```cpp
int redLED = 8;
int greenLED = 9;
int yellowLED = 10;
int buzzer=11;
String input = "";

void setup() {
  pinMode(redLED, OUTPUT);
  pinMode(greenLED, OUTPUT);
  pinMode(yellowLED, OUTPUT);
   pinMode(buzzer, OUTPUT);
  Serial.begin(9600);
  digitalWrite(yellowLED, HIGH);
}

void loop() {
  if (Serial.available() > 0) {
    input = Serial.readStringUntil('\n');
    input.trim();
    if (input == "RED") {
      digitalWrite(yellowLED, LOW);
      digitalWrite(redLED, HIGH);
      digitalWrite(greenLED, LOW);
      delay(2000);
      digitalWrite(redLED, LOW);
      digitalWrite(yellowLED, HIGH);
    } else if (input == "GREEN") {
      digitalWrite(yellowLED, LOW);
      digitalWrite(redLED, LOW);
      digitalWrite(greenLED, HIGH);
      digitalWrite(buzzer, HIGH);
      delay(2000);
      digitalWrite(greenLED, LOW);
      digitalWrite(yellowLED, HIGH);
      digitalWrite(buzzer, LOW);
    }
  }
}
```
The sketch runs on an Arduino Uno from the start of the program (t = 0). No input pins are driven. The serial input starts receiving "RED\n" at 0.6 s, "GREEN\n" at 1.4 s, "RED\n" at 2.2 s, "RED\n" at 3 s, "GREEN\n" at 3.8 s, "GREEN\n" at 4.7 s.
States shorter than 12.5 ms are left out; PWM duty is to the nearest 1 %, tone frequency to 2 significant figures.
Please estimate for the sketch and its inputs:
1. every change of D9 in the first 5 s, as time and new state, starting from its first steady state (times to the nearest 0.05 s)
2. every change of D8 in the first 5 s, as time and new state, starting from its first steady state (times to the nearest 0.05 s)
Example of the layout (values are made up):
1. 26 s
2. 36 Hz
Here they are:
1. 0 s low; 2.6 s high; 4.6 s low
2. 0 s low; 0.6 s high; 2.6 s low; 4.6 s high
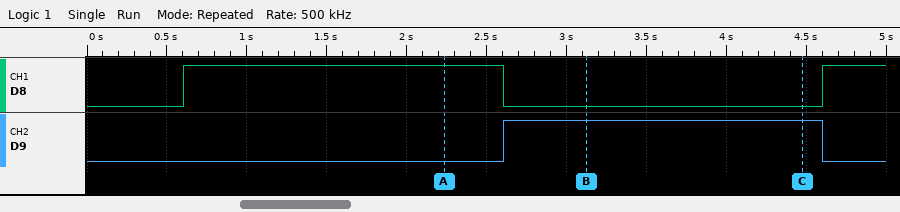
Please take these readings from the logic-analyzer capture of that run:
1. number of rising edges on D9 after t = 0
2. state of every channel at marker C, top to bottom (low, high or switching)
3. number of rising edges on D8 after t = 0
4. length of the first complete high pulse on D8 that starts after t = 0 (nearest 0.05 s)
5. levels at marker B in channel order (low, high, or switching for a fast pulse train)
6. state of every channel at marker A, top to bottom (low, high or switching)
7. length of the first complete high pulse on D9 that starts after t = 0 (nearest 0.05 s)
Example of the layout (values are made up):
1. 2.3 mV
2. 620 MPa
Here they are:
1. 1
2. D8 low, D9 high
3. 2
4. 2.00 s
5. D8 low, D9 high
6. D8 high, D9 low
7. 2.00 s
